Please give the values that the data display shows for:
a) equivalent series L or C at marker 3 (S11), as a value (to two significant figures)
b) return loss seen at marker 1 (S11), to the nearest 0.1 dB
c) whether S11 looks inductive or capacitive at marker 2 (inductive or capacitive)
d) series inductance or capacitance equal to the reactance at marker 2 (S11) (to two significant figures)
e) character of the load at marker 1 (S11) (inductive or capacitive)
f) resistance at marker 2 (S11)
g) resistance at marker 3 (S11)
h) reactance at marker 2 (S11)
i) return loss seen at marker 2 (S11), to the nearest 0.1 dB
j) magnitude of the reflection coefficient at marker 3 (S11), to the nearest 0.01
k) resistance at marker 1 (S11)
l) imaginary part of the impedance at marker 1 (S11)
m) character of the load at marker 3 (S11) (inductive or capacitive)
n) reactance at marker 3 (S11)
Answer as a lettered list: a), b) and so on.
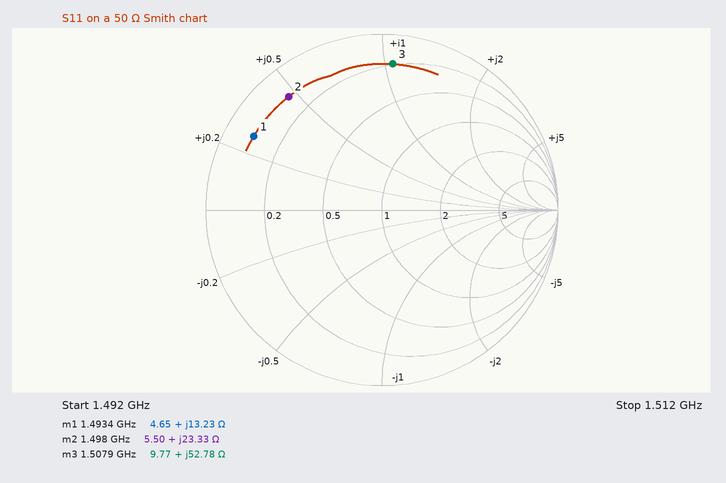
a) 5.6 nH
b) 1.5 dB
c) inductive
d) 2.5 nH
e) inductive
f) 5.50 Ω
g) 9.77 Ω
h) +23.33 Ω
i) 1.6 dB
j) 0.83
k) 4.65 Ω
l) +13.23 Ω
m) inductive
n) +52.78 Ω
